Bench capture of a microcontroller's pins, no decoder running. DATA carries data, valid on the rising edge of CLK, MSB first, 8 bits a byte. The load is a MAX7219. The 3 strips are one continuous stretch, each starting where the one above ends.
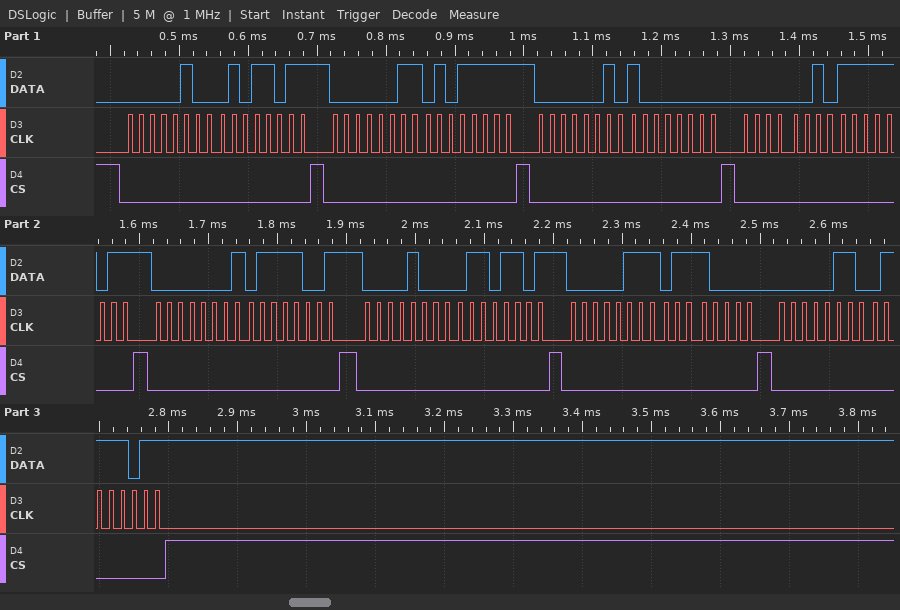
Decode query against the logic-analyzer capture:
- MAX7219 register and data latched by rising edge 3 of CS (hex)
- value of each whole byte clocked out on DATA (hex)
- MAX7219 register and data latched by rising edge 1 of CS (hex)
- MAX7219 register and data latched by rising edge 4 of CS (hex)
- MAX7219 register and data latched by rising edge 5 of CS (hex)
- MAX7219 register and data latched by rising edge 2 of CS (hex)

register 0x2, data 0x80
04 5B 03 5F 02 80 02 FB 01 79 08 6D 07 70 06 7B
register 0x4, data 0x5B
register 0x2, data 0xFB
register 0x1, data 0x79
register 0x3, data 0x5F
